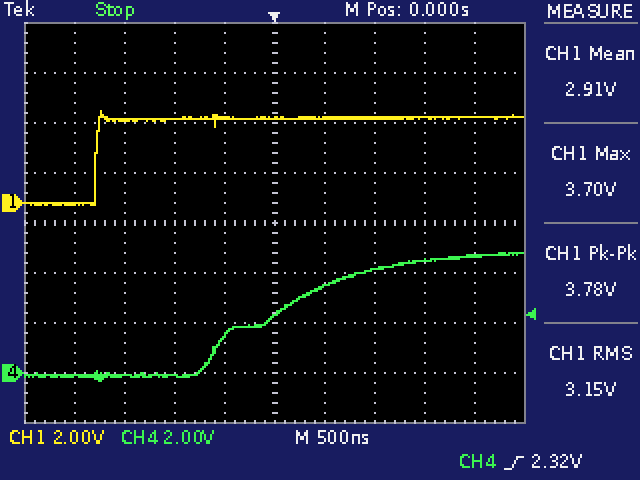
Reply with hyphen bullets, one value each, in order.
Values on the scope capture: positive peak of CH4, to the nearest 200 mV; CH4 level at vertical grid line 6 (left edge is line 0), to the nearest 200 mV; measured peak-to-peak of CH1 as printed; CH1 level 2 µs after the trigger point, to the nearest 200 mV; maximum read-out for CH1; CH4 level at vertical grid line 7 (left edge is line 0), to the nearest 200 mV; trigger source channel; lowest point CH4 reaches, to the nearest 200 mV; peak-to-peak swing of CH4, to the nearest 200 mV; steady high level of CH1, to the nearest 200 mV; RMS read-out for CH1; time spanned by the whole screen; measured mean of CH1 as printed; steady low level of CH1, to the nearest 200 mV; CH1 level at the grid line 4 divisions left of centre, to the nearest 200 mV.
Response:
- 4.8 V
- 3.4 V
- 3.78 V
- 3.4 V
- 3.70 V
- 4.2 V
- CH4
- -400 mV
- 5.2 V
- 3.4 V
- 3.15 V
- 5 µs
- 2.91 V
- 0.0 V
- 0.0 V
